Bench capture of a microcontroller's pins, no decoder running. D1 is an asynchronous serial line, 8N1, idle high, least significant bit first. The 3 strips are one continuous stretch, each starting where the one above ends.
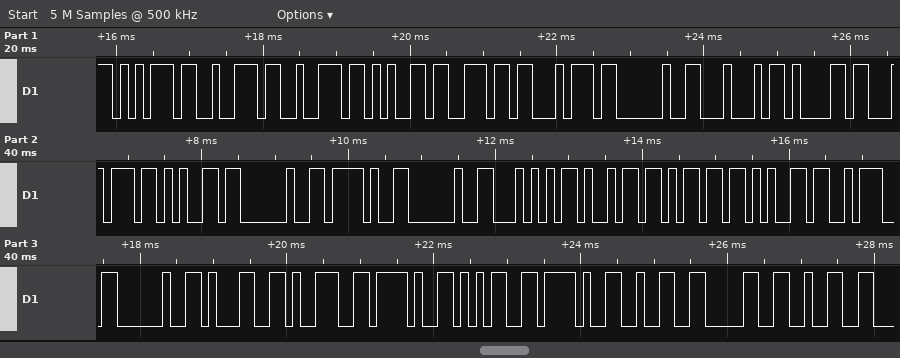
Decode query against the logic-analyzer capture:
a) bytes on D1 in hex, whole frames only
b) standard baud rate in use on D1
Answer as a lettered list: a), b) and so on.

a) 75 72 72 65 6E 74 20 44 61 74 65 20 2F 20 54 69 6D 65 3A 20 31 39 2F 35 2F 32 30 32
b) 9600 baud
